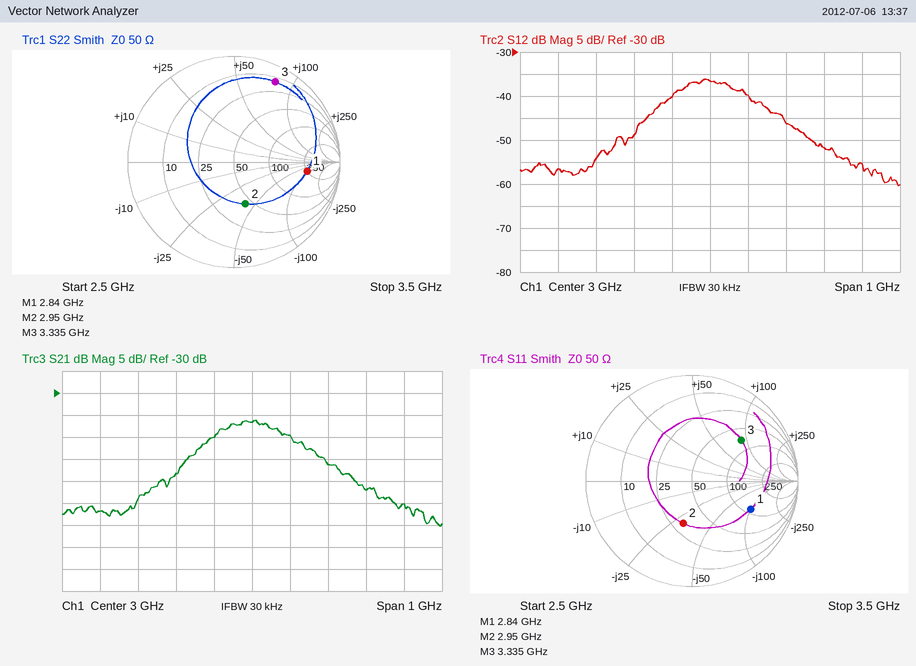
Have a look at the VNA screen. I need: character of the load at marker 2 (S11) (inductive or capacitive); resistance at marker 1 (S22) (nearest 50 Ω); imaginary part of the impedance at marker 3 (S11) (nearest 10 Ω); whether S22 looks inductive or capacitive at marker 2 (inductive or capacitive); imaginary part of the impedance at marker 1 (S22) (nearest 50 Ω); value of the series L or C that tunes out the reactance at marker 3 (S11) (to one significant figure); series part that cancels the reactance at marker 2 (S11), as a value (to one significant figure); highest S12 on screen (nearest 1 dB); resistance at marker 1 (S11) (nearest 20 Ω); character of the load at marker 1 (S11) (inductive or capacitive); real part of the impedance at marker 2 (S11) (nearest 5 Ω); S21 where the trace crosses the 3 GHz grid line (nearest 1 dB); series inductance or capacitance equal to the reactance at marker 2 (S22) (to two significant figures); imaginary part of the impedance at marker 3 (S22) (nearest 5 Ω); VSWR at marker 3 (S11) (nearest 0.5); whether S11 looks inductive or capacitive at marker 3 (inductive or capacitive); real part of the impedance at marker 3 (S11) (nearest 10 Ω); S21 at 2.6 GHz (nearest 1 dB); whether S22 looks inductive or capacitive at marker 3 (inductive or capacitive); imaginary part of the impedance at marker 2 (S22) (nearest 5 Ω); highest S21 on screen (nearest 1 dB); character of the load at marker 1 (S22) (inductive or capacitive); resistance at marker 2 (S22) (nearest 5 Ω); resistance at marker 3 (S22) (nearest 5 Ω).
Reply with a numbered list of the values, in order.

1. capacitive
2. 250 Ω
3. +90 Ω
4. capacitive
5. -100 Ω
6. 500 fF
7. 2 nH
8. -36 dB
9. 120 Ω
10. capacitive
11. 30 Ω
12. -37 dB
13. 1.3 pF
14. +80 Ω
15. 4.0
16. inductive
17. 70 Ω
18. -57 dB
19. inductive
20. -40 Ω
21. -36 dB
22. capacitive
23. 45 Ω
24. 15 Ω
